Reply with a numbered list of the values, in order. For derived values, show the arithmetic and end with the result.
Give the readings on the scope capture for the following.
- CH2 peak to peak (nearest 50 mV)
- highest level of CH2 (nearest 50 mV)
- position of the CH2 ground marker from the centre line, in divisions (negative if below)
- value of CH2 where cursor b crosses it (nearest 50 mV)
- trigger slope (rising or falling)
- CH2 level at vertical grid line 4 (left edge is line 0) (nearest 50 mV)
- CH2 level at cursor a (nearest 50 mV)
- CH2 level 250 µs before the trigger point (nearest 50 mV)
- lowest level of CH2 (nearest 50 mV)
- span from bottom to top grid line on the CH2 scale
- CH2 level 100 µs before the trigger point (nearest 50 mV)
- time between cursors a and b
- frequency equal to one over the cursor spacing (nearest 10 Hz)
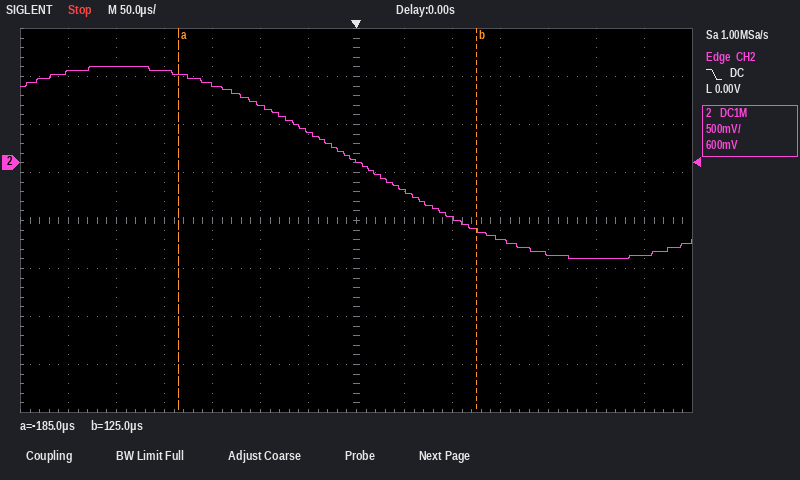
1. 1.00 V − (-1.00 V) = 2.00 V
2. 1.00 V
3. +1.2 div
4. -700 mV
5. falling
6. 800 mV
7. 900 mV
8. 1.00 V
9. -1.00 V
10. 4 V
11. 600 mV
12. 125 µs − (-185 µs) = 310 µs
13. 1 / 310 µs ≈ 3.23 kHz
